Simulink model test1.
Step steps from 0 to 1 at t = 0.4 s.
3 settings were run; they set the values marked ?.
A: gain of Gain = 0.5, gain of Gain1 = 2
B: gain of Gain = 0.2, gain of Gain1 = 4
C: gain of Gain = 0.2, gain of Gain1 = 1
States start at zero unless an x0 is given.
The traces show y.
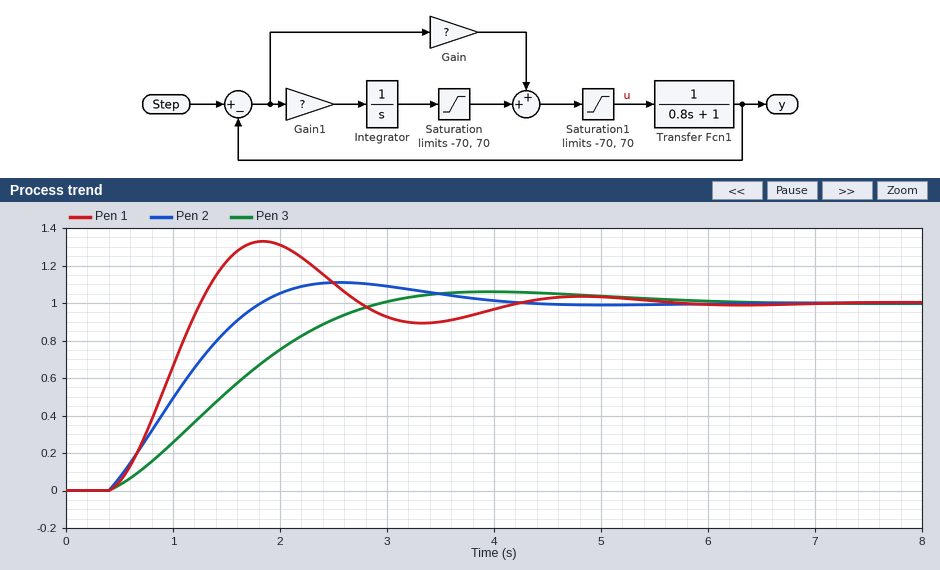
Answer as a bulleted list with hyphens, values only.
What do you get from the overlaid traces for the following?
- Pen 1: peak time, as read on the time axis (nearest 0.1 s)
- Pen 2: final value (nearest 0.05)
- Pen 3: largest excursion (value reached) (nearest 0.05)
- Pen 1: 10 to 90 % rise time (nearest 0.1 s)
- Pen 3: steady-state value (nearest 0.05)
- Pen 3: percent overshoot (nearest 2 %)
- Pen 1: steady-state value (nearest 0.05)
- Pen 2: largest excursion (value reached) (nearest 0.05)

- 1.8 s
- 1.00
- 1.05
- 0.6 s
- 1.00
- 6 %
- 1.00
- 1.10
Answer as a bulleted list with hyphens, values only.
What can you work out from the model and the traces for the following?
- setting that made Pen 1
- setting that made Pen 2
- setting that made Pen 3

- B
- A
- C
